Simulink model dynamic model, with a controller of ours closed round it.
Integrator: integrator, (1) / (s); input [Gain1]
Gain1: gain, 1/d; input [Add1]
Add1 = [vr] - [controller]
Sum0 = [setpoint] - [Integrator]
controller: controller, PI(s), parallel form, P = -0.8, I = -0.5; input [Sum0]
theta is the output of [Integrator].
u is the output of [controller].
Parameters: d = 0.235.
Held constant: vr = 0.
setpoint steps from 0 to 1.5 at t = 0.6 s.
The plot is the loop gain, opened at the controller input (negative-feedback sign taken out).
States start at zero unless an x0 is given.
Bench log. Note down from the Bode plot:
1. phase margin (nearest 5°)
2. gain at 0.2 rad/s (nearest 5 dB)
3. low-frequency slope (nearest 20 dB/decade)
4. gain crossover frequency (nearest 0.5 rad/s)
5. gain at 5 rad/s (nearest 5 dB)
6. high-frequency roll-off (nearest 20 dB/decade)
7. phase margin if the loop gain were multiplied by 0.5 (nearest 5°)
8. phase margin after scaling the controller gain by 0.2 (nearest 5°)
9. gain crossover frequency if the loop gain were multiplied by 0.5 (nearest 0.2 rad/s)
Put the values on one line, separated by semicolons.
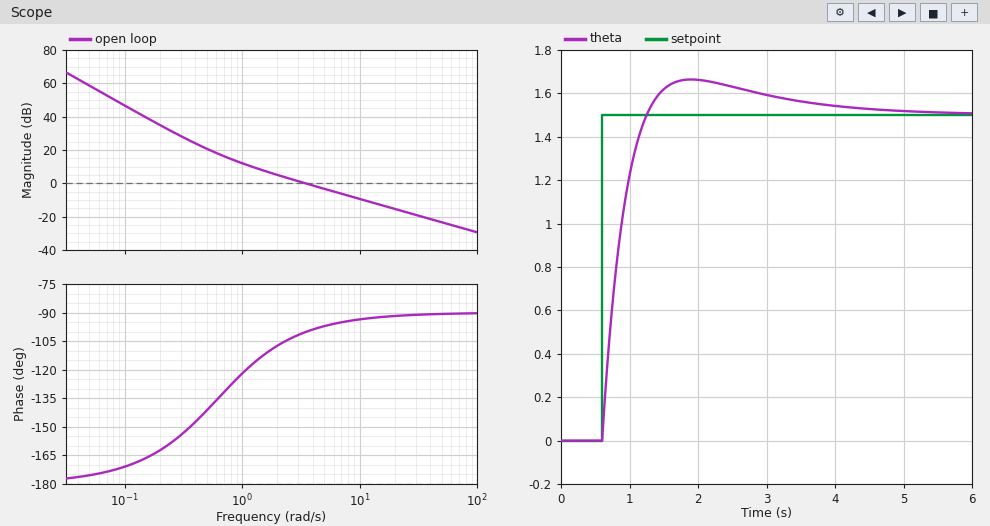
80°; 35 dB; -40 dB/decade; 3.5 rad/s; -5 dB; -20 dB/decade; 70°; 55°; 1.8 rad/s
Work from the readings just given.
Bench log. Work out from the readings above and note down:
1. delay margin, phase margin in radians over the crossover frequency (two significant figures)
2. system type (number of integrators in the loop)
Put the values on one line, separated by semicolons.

0.40 s; 2
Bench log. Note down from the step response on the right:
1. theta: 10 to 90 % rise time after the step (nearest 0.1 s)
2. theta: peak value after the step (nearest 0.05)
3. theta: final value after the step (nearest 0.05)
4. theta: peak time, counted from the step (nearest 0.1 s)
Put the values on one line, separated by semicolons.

0.5 s; 1.65; 1.50; 1.3 s
